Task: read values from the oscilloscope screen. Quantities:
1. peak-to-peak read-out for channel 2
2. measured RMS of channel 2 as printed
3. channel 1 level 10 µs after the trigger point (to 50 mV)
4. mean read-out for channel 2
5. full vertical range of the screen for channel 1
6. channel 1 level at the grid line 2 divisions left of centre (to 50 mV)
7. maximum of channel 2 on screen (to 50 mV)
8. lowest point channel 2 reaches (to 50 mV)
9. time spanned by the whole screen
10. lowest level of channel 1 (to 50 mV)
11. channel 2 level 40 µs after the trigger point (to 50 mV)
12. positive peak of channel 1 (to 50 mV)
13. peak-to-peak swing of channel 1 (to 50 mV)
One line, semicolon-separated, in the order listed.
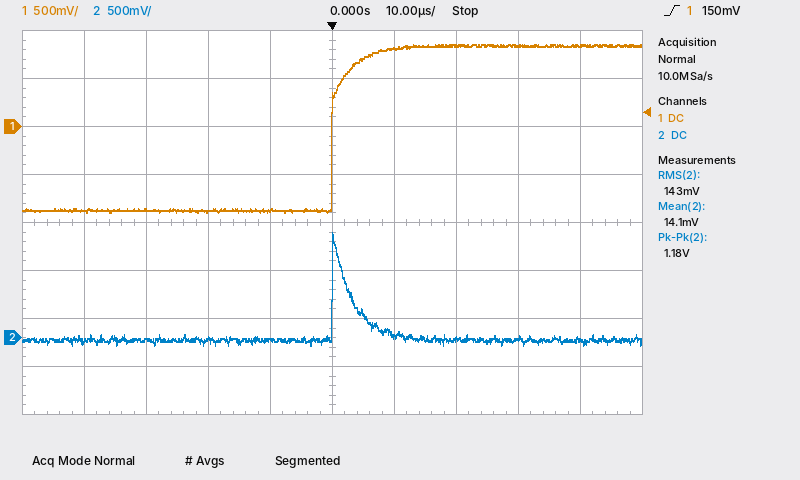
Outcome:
1.18 V; 143 mV; 800 mV; 14.1 mV; 4 V; -900 mV; 1.10 V; -100 mV; 100 µs; -900 mV; 0 mV; 850 mV; 1.75 V
